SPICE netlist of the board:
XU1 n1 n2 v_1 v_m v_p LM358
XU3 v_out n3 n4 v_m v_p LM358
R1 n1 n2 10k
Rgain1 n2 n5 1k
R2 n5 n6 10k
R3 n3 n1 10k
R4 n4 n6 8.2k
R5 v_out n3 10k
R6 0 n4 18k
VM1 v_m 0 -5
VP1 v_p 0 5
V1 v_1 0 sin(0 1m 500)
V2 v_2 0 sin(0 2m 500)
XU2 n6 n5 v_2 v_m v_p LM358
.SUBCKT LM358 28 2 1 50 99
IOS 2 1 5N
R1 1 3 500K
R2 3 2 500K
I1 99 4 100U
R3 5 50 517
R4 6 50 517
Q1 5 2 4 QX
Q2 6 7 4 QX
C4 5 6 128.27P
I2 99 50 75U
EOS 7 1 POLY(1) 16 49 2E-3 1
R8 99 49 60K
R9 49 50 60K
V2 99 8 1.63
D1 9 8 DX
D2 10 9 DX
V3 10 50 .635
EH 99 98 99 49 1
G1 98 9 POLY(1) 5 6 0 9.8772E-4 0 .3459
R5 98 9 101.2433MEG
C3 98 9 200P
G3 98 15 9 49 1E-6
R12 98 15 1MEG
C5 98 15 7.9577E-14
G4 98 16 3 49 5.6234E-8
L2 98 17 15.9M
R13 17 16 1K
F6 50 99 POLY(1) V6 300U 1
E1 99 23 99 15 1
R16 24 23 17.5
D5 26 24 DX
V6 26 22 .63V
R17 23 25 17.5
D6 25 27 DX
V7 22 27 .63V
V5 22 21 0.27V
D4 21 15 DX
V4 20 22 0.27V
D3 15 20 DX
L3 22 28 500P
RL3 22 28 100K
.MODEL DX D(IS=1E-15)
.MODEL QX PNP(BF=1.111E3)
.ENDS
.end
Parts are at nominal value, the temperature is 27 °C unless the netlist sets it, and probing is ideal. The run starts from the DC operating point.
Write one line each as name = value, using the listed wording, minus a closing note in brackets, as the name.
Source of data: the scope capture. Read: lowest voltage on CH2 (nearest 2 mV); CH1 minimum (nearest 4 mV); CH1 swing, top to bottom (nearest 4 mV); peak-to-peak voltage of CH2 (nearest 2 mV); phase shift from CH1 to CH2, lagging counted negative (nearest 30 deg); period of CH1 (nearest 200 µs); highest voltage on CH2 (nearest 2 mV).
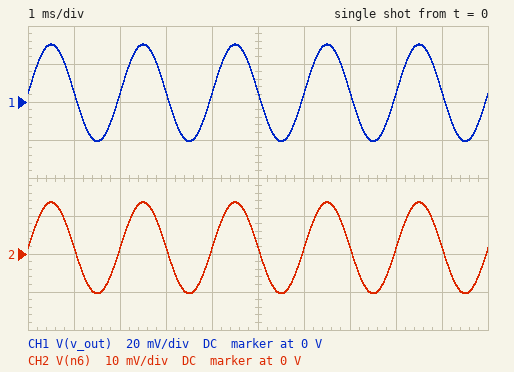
lowest voltage on CH2 = -10 mV
CH1 minimum = -20 mV
CH1 swing, top to bottom = 52 mV
peak-to-peak voltage of CH2 = 24 mV
phase shift from CH1 to CH2, lagging counted negative = 0 deg
period of CH1 = 2.0 ms
highest voltage on CH2 = 14 mV
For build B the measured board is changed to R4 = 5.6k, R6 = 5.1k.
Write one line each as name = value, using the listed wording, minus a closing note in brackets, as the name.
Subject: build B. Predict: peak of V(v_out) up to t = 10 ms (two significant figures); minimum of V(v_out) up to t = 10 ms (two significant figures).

peak of V(v_out) up to t = 10 ms = 24 mV
minimum of V(v_out) up to t = 10 ms = -17 mV
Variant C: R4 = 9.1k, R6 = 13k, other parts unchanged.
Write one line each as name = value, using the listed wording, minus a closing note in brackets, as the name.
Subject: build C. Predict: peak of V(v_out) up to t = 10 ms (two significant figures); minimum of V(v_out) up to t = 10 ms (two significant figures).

peak of V(v_out) up to t = 10 ms = 28 mV
minimum of V(v_out) up to t = 10 ms = -19 mV
